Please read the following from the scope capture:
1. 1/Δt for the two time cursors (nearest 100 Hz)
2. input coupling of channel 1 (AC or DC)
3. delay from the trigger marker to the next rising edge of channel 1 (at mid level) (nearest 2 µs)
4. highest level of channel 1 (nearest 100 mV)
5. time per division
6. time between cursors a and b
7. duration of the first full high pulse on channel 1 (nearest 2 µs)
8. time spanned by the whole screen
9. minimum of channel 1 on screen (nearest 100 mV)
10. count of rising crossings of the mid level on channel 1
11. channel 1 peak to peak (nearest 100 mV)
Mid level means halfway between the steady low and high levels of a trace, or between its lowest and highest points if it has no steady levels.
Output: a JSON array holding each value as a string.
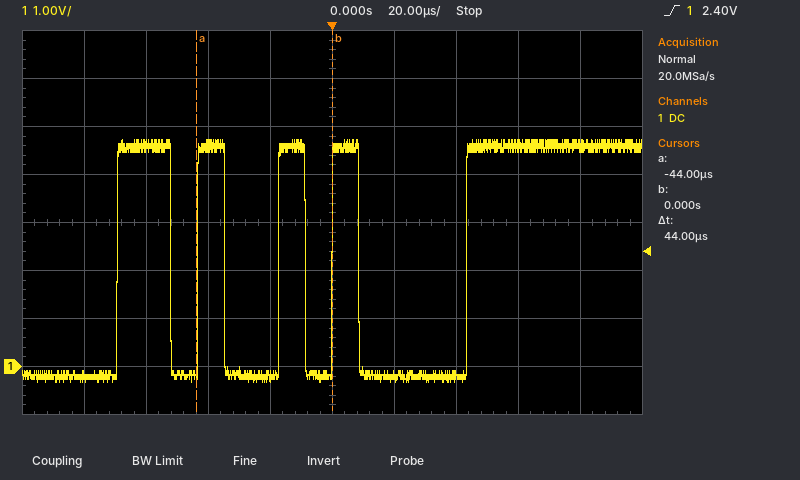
["22.7 kHz", "DC", "44 µs", "4.7 V", "20 µs", "44 µs", "18 µs", "200 µs", "-300 mV", "5", "5.0 V"]
